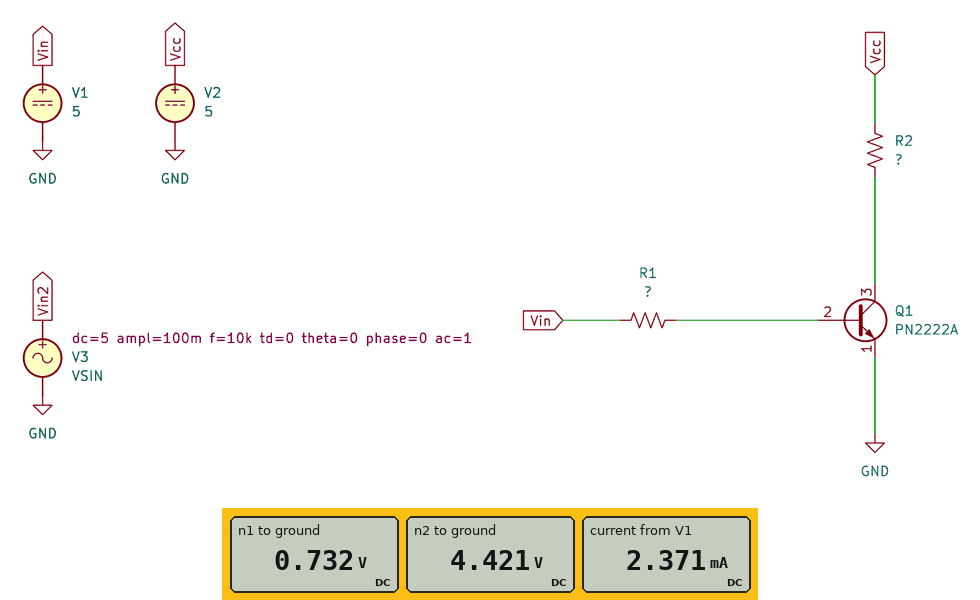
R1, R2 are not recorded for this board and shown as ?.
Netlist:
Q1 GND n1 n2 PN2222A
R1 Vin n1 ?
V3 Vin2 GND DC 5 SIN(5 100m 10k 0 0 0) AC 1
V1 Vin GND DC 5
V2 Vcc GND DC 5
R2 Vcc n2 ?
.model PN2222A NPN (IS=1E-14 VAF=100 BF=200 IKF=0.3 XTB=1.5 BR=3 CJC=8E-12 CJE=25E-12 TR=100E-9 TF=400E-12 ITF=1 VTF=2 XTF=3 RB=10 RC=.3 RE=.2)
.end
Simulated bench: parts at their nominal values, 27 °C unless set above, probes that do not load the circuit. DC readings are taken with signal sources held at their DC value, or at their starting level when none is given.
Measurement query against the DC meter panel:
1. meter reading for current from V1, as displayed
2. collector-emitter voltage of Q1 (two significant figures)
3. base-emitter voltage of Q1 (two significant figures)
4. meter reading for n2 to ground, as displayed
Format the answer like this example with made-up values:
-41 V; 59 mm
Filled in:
2.371 mA; -4.4 V; -3.7 V; 4.421 V
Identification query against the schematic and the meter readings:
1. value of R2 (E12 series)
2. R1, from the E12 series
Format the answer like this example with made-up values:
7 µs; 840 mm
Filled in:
82 Ω; 1.8 kΩ
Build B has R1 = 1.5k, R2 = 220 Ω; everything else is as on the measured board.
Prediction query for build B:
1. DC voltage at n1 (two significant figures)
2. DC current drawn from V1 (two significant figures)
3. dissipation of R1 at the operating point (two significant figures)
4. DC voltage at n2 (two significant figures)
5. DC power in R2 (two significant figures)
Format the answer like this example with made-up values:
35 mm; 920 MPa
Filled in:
740 mV; 2.8 mA; 12 mW; 3.1 V; 16 mW
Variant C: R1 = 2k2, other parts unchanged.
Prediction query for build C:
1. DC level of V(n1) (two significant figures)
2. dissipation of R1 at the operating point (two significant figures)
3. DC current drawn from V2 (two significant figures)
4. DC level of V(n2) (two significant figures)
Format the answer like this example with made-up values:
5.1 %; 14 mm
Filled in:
720 mV; 8.3 mW; 5.8 mA; 4.5 V
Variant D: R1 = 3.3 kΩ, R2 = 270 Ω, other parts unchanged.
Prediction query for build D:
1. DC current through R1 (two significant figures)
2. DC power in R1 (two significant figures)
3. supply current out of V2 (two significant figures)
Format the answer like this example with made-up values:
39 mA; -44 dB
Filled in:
1.3 mA; 5.6 mW; 3.9 mA
